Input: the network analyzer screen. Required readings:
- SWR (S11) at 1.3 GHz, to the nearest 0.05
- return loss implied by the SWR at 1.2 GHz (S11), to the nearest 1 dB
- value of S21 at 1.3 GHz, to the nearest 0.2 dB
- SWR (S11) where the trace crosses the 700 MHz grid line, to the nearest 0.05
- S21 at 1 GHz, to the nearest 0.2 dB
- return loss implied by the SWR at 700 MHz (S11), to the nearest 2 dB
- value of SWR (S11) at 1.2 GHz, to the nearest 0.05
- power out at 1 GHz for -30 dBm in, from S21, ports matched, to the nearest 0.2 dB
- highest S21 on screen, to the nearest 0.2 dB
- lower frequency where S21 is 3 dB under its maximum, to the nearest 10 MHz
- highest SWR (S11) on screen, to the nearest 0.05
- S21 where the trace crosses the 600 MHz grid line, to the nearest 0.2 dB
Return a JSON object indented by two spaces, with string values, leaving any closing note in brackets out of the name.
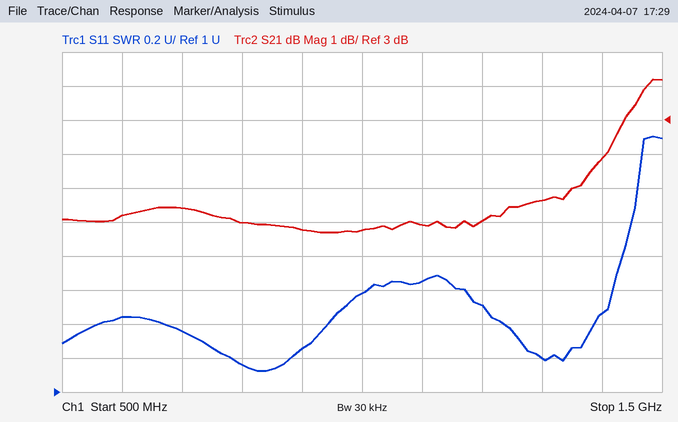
{
  "SWR (S11) at 1.3 GHz, to the nearest 0.05": "1.20",
  "return loss implied by the SWR at 1.2 GHz (S11), to the nearest 1 dB": "14 dB",
  "value of S21 at 1.3 GHz, to the nearest 0.2 dB": "0.6 dB",
  "SWR (S11) where the trace crosses the 700 MHz grid line, to the nearest 0.05": "1.35",
  "S21 at 1 GHz, to the nearest 0.2 dB": "-0.2 dB",
  "return loss implied by the SWR at 700 MHz (S11), to the nearest 2 dB": "16 dB",
  "value of SWR (S11) at 1.2 GHz, to the nearest 0.05": "1.50",
  "power out at 1 GHz for -30 dBm in, from S21, ports matched, to the nearest 0.2 dB": "-30.2 dBm",
  "highest S21 on screen, to the nearest 0.2 dB": "4.2 dB",
  "lower frequency where S21 is 3 dB under its maximum, to the nearest 10 MHz": "1.37 GHz",
  "highest SWR (S11) on screen, to the nearest 0.05": "2.50",
  "S21 where the trace crosses the 600 MHz grid line, to the nearest 0.2 dB": "0.2 dB"
}
